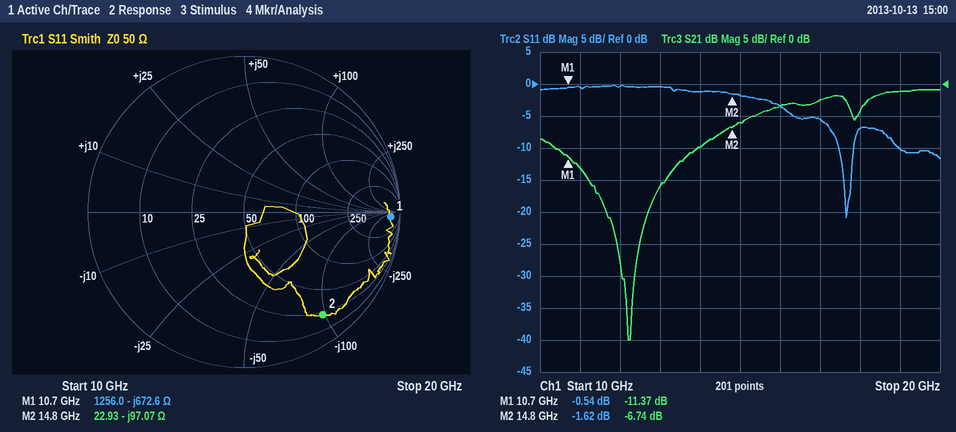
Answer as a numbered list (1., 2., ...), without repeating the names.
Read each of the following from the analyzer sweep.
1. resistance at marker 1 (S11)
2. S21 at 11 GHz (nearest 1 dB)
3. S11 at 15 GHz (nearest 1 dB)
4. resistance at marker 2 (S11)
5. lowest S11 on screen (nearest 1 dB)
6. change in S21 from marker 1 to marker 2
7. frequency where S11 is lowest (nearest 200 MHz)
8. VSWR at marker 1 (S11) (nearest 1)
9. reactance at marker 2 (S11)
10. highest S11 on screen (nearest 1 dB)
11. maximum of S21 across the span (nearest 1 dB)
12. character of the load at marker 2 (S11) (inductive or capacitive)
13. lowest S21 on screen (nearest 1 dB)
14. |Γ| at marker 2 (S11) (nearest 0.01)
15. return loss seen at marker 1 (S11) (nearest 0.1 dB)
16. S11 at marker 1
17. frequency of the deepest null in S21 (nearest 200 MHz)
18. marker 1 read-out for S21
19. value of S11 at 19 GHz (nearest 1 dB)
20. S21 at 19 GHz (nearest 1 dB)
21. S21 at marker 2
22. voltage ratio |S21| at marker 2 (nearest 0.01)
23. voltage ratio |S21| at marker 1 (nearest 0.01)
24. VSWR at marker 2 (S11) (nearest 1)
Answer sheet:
1. 1256.0 Ω
2. -13 dB
3. -2 dB
4. 22.93 Ω
5. -21 dB
6. 4.63 dB
7. 17.6 GHz
8. 32
9. -97.07 Ω
10. 0 dB
11. -1 dB
12. capacitive
13. -40 dB
14. 0.83
15. 0.5 dB
16. -0.54 dB
17. 12.2 GHz
18. -11.37 dB
19. -10 dB
20. -1 dB
21. -6.74 dB
22. 0.46
23. 0.27
24. 11
